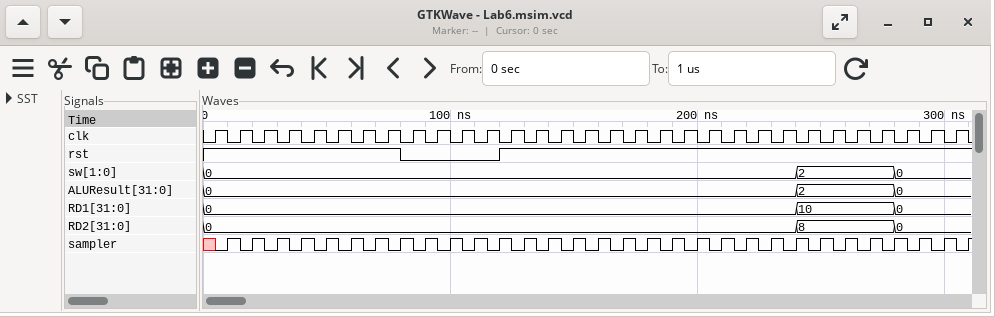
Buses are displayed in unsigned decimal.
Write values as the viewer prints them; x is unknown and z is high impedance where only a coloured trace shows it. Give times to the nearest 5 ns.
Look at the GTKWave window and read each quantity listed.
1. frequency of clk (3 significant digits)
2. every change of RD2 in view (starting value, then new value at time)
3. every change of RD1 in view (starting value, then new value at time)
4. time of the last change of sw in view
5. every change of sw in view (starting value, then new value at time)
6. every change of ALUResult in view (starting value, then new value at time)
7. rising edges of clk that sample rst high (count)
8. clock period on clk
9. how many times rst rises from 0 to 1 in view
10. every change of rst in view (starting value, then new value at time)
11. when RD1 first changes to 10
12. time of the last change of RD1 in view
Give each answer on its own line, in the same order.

100 MHz
0, 8 at 240 ns, 0 at 280 ns
0, 10 at 240 ns, 0 at 280 ns
280 ns
0, 2 at 240 ns, 0 at 280 ns
0, 2 at 240 ns, 0 at 280 ns
27
10 ns
1
1, 0 at 80 ns, 1 at 120 ns
240 ns
280 ns
